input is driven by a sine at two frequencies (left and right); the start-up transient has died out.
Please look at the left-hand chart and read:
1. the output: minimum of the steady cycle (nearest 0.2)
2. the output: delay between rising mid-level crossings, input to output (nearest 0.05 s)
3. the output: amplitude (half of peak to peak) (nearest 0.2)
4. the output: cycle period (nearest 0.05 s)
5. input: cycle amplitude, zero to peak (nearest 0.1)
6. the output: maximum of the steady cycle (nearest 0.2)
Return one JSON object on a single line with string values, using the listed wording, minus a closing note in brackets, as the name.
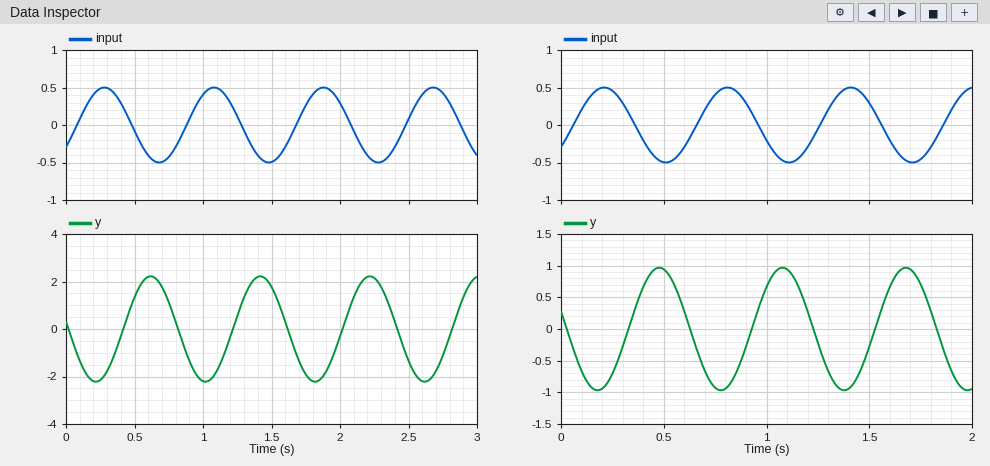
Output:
{"the output: minimum of the steady cycle": "-2.2", "the output: delay between rising mid-level crossings, input to output": "0.35 s", "the output: amplitude (half of peak to peak)": "2.2", "the output: cycle period": "0.80 s", "input: cycle amplitude, zero to peak": "0.5", "the output: maximum of the steady cycle": "2.2"}
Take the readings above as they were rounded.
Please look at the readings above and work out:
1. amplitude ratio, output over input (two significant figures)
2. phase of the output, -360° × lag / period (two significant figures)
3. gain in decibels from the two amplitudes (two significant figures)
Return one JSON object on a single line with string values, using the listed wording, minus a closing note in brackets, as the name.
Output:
{"amplitude ratio, output over input": "4.4", "phase of the output, -360° × lag / period": "-160°", "gain in decibels from the two amplitudes": "13 dB"}
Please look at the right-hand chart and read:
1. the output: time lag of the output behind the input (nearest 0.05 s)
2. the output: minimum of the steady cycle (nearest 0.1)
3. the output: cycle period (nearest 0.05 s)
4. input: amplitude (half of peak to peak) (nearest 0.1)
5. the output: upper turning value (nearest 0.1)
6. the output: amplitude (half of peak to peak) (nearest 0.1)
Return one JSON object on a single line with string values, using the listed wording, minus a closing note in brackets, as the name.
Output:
{"the output: time lag of the output behind the input": "0.25 s", "the output: minimum of the steady cycle": "-1.0", "the output: cycle period": "0.60 s", "input: amplitude (half of peak to peak)": "0.5", "the output: upper turning value": "1.0", "the output: amplitude (half of peak to peak)": "1.0"}
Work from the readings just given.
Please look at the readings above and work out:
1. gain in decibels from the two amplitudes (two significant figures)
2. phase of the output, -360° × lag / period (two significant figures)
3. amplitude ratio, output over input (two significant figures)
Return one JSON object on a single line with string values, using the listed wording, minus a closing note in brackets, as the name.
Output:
{"gain in decibels from the two amplitudes": "6.0 dB", "phase of the output, -360° × lag / period": "-150°", "amplitude ratio, output over input": "2.0"}
